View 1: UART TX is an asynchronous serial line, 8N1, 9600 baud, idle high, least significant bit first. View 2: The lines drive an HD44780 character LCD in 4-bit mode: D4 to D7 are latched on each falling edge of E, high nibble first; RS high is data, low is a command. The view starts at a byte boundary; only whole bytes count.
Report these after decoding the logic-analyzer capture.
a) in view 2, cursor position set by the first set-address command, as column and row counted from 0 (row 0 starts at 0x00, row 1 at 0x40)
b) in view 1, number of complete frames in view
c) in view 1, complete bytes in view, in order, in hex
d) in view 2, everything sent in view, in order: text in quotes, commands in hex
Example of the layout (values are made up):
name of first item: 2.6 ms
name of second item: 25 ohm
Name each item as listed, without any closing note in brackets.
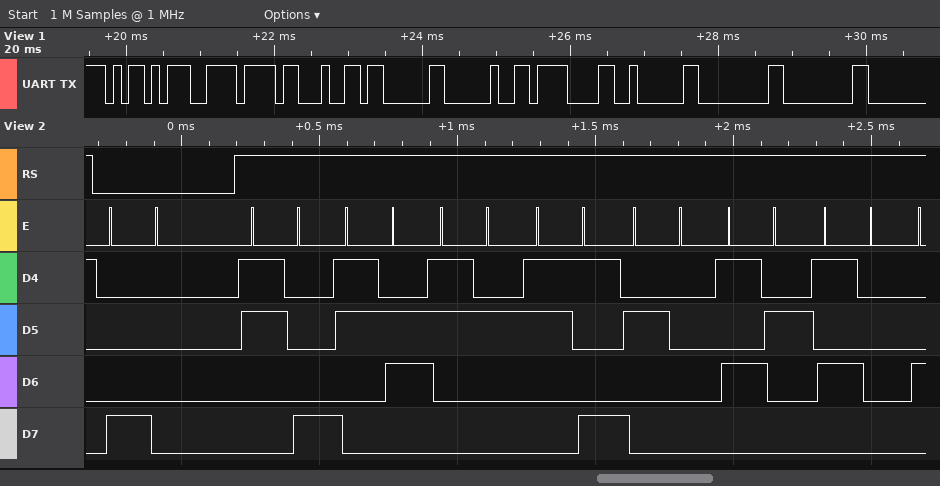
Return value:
in view 2, cursor position set by the first set-address command, as column and row counted from 0: column 0, row 0
in view 1, number of complete frames in view: 9
in view 1, complete bytes in view, in order, in hex: AD DE 23 03 20 0F 02 00 00
in view 2, everything sent in view, in order: text in quotes, commands in hex: 0x80 "8629 RP"
